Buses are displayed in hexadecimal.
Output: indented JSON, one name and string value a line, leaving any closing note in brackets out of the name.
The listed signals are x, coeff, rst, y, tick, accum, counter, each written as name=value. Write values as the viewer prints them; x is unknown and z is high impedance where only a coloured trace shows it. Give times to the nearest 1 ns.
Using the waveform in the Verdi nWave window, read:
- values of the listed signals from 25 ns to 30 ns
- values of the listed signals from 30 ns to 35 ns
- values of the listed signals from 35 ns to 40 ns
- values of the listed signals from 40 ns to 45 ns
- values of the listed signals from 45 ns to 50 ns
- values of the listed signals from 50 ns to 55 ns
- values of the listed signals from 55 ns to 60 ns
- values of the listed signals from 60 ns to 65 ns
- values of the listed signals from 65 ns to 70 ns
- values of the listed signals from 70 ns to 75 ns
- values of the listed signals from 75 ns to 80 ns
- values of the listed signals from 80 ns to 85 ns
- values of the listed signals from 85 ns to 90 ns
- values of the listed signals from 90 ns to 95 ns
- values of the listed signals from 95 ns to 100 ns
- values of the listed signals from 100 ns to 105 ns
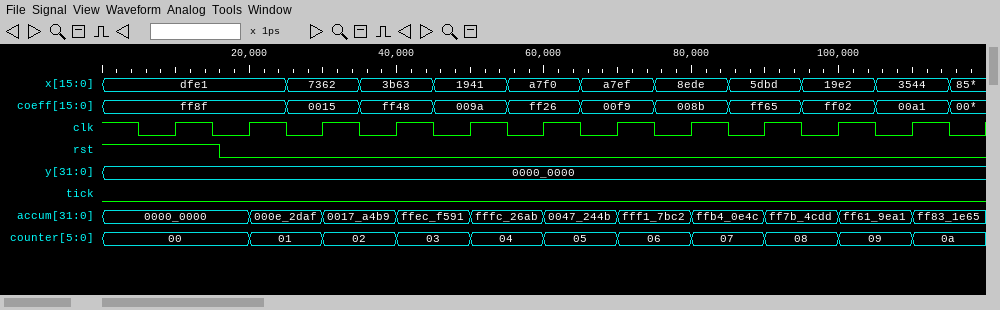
{
  "values of the listed signals from 25 ns to 30 ns": "x=7362, coeff=0015, rst=0, y=0000_0000, tick=0, accum=000e_2daf, counter=01",
  "values of the listed signals from 30 ns to 35 ns": "x=7362, coeff=0015, rst=0, y=0000_0000, tick=0, accum=0017_a4b9, counter=02",
  "values of the listed signals from 35 ns to 40 ns": "x=3b63, coeff=ff48, rst=0, y=0000_0000, tick=0, accum=0017_a4b9, counter=02",
  "values of the listed signals from 40 ns to 45 ns": "x=3b63, coeff=ff48, rst=0, y=0000_0000, tick=0, accum=ffec_f591, counter=03",
  "values of the listed signals from 45 ns to 50 ns": "x=1941, coeff=009a, rst=0, y=0000_0000, tick=0, accum=ffec_f591, counter=03",
  "values of the listed signals from 50 ns to 55 ns": "x=1941, coeff=009a, rst=0, y=0000_0000, tick=0, accum=fffc_26ab, counter=04",
  "values of the listed signals from 55 ns to 60 ns": "x=a7f0, coeff=ff26, rst=0, y=0000_0000, tick=0, accum=fffc_26ab, counter=04",
  "values of the listed signals from 60 ns to 65 ns": "x=a7f0, coeff=ff26, rst=0, y=0000_0000, tick=0, accum=0047_244b, counter=05",
  "values of the listed signals from 65 ns to 70 ns": "x=a7ef, coeff=00f9, rst=0, y=0000_0000, tick=0, accum=0047_244b, counter=05",
  "values of the listed signals from 70 ns to 75 ns": "x=a7ef, coeff=00f9, rst=0, y=0000_0000, tick=0, accum=fff1_7bc2, counter=06",
  "values of the listed signals from 75 ns to 80 ns": "x=8ede, coeff=008b, rst=0, y=0000_0000, tick=0, accum=fff1_7bc2, counter=06",
  "values of the listed signals from 80 ns to 85 ns": "x=8ede, coeff=008b, rst=0, y=0000_0000, tick=0, accum=ffb4_0e4c, counter=07",
  "values of the listed signals from 85 ns to 90 ns": "x=5dbd, coeff=ff65, rst=0, y=0000_0000, tick=0, accum=ffb4_0e4c, counter=07",
  "values of the listed signals from 90 ns to 95 ns": "x=5dbd, coeff=ff65, rst=0, y=0000_0000, tick=0, accum=ff7b_4cdd, counter=08",
  "values of the listed signals from 95 ns to 100 ns": "x=19e2, coeff=ff02, rst=0, y=0000_0000, tick=0, accum=ff7b_4cdd, counter=08",
  "values of the listed signals from 100 ns to 105 ns": "x=19e2, coeff=ff02, rst=0, y=0000_0000, tick=0, accum=ff61_9ea1, counter=09"
}
